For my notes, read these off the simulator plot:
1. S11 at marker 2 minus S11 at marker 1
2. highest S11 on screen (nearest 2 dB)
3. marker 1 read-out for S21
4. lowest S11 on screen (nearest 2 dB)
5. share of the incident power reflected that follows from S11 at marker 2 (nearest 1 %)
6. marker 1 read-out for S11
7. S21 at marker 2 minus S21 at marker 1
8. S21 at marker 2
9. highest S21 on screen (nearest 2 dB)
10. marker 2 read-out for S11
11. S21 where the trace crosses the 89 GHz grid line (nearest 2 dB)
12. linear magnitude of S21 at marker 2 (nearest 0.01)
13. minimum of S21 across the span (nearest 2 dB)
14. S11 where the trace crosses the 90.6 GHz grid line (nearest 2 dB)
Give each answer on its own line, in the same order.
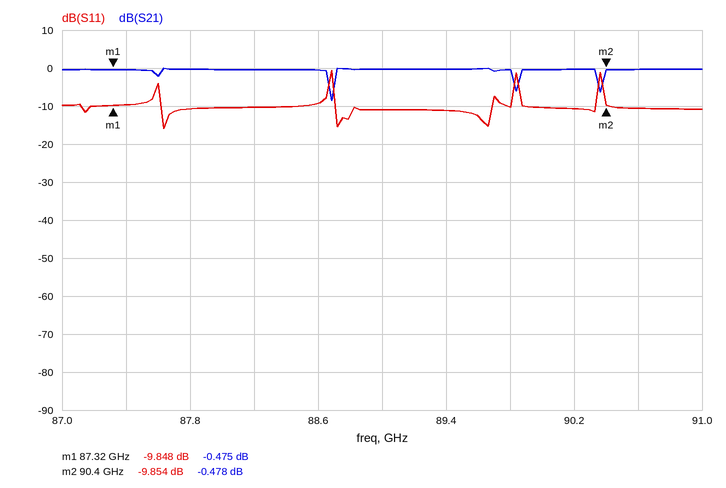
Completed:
-0.006 dB
0 dB
-0.475 dB
-16 dB
10 %
-9.848 dB
-0.003 dB
-0.478 dB
0 dB
-9.854 dB
0 dB
0.95
-8 dB
-10 dB
